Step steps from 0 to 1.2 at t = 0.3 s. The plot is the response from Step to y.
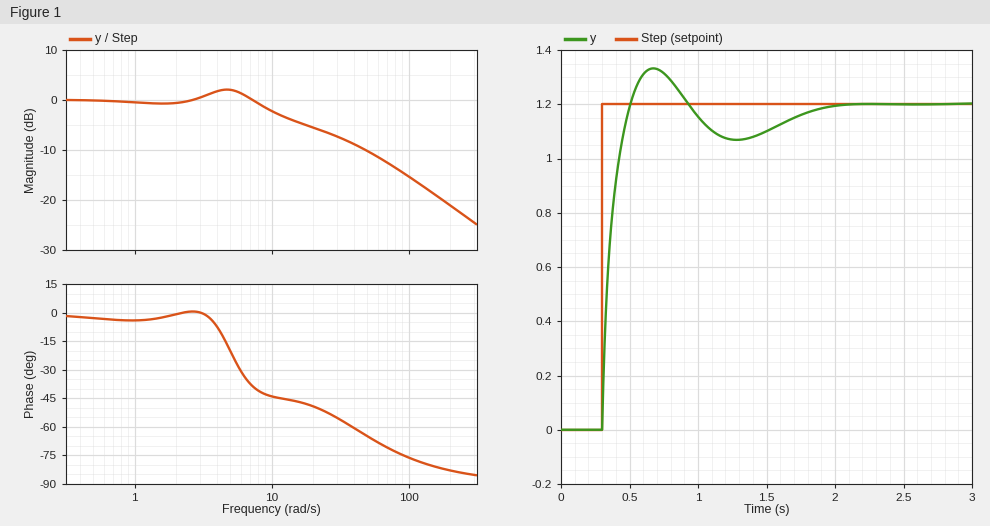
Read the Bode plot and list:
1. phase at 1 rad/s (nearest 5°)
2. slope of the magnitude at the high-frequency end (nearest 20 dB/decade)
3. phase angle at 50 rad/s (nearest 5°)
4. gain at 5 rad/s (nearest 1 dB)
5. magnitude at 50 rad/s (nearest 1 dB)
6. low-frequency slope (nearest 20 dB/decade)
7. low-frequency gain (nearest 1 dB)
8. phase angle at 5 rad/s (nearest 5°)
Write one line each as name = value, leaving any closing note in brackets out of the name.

phase at 1 rad/s = -5°
slope of the magnitude at the high-frequency end = -20 dB/decade
phase angle at 50 rad/s = -65°
gain at 5 rad/s = 2 dB
magnitude at 50 rad/s = -10 dB
low-frequency slope = 0 dB/decade
low-frequency gain = 0 dB
phase angle at 5 rad/s = -20°
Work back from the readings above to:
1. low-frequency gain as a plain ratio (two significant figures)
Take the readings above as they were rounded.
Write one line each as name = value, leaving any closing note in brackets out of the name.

low-frequency gain as a plain ratio = 1.0
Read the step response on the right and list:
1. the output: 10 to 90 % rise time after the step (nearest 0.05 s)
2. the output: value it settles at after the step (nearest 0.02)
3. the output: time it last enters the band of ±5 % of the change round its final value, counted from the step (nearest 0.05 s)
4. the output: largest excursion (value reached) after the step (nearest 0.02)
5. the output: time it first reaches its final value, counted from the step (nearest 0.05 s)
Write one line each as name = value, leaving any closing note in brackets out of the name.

the output: 10 to 90 % rise time after the step = 0.15 s
the output: value it settles at after the step = 1.20
the output: time it last enters the band of ±5 % of the change round its final value, counted from the step = 1.35 s
the output: largest excursion (value reached) after the step = 1.34
the output: time it first reaches its final value, counted from the step = 0.20 s
